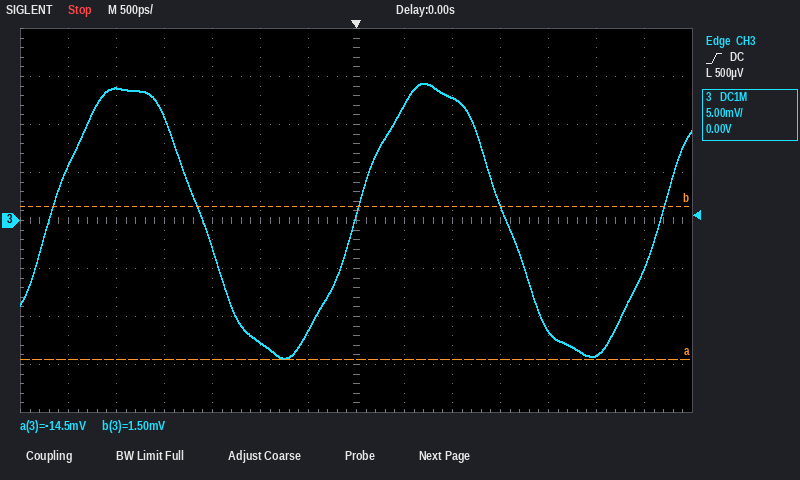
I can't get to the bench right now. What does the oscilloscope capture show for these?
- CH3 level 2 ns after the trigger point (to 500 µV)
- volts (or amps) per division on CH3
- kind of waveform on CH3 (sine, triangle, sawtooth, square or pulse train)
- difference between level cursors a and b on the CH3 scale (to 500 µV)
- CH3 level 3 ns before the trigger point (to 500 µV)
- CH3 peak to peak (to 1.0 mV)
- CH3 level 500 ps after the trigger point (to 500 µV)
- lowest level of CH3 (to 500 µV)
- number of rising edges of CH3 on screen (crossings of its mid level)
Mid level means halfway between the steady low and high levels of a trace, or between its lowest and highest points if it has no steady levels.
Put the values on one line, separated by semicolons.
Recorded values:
-11.5 mV; 5 mV; sine; 16.0 mV; 5.5 mV; 29.0 mV; 12.0 mV; -14.5 mV; 3
